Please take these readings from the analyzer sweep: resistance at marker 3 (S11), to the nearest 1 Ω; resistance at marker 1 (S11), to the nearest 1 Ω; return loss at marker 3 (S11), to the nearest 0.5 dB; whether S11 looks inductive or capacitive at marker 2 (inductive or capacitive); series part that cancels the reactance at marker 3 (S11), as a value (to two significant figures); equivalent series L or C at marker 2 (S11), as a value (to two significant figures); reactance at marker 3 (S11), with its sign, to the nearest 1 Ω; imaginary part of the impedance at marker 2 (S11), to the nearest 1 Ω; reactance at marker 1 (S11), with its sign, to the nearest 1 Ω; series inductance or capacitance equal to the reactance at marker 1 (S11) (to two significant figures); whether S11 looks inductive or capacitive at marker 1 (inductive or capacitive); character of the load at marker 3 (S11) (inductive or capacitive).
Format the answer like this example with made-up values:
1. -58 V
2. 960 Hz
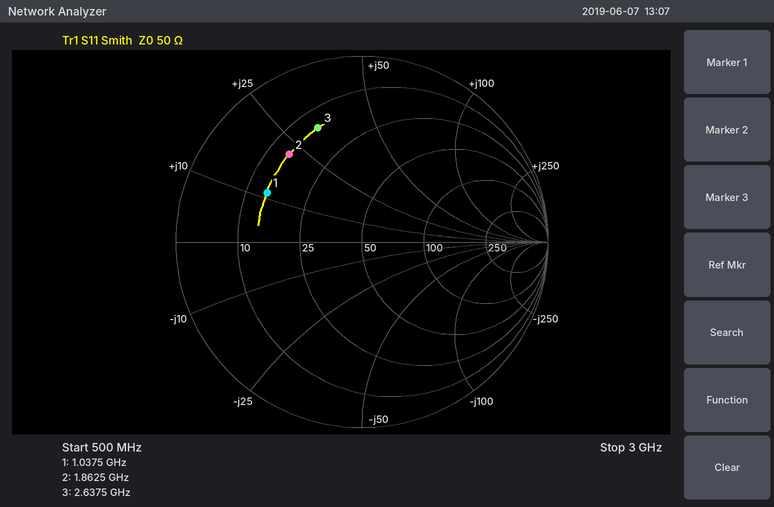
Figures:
1. 15 Ω
2. 14 Ω
3. 3.5 dB
4. inductive
5. 1.9 pF
6. 1.9 nH
7. +32 Ω
8. +22 Ω
9. +11 Ω
10. 1.7 nH
11. inductive
12. inductive
